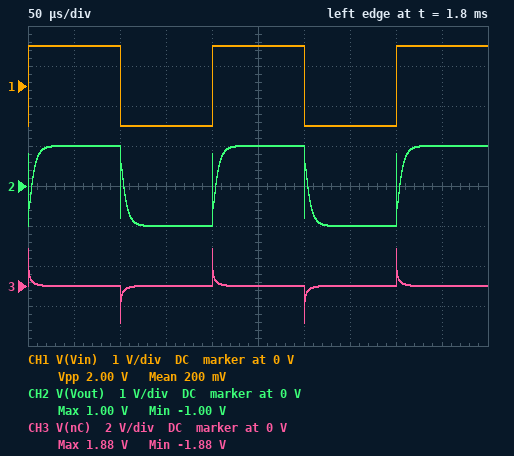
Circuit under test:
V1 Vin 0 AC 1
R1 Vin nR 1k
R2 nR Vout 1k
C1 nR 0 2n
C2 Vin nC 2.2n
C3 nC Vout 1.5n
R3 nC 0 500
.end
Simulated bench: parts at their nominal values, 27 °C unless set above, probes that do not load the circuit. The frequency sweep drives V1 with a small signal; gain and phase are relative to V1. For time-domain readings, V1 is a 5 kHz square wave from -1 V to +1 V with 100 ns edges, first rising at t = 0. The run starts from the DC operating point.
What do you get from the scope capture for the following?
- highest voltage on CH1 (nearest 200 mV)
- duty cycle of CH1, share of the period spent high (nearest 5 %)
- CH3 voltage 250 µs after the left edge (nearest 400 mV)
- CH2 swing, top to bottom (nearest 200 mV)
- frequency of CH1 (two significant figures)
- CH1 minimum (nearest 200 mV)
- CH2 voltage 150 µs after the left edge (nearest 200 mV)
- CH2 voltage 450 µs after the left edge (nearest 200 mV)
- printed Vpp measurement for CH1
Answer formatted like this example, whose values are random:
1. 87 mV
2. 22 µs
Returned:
1. 1.0 V
2. 50 %
3. 0 V
4. 2.0 V
5. 5.0 kHz
6. -1.0 V
7. -1.0 V
8. 1.0 V
9. 2.00 V
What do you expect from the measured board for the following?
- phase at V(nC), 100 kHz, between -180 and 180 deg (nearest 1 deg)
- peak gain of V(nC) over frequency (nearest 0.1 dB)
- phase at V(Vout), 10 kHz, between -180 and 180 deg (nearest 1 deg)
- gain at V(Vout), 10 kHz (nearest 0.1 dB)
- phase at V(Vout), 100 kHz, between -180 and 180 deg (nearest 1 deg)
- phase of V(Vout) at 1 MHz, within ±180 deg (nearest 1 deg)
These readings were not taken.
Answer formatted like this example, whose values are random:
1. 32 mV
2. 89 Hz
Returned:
1. 41 deg
2. 0 dB
3. -17 deg
4. -0.5 dB
5. 1 deg
6. 18 deg
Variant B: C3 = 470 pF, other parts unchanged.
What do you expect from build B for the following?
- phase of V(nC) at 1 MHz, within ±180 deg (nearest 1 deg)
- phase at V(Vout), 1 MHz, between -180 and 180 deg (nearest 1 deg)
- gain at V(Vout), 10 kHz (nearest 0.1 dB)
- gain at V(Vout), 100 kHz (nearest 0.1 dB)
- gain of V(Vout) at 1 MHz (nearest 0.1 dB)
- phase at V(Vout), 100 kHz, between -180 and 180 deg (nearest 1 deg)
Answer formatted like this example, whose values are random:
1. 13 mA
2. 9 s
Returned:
1. 11 deg
2. 29 deg
3. -0.2 dB
4. -9.8 dB
5. -1.3 dB
6. -64 deg
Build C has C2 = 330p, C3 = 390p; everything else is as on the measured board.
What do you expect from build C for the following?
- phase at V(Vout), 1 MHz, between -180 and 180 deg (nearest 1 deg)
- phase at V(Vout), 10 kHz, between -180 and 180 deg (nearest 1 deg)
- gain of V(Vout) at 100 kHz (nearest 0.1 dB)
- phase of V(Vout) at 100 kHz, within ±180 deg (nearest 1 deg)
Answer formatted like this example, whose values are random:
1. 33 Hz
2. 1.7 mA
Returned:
1. 71 deg
2. -10 deg
3. -6.2 dB
4. -68 deg
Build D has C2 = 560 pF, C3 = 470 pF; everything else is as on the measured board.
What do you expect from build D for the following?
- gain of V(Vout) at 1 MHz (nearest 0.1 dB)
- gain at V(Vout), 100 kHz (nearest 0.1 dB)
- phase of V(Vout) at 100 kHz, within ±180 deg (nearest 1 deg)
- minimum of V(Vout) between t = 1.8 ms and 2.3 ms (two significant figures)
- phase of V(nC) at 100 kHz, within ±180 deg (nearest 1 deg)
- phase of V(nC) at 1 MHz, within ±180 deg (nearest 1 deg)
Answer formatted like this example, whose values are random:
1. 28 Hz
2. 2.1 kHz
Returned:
1. -3.8 dB
2. -7.1 dB
3. -71 deg
4. -1.0 V
5. 55 deg
6. 36 deg
